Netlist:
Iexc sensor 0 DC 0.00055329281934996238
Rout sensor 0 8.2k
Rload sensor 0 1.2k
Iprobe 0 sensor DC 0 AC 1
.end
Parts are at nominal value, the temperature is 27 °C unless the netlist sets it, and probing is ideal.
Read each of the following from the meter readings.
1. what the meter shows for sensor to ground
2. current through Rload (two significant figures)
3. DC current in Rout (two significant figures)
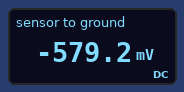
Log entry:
-579.2 mV
480 µA
71 µA
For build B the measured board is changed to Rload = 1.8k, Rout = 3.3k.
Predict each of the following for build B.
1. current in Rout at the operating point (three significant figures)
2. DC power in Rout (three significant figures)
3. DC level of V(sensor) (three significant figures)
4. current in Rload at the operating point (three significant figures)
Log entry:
195 µA
126 µW
-644 mV
358 µA
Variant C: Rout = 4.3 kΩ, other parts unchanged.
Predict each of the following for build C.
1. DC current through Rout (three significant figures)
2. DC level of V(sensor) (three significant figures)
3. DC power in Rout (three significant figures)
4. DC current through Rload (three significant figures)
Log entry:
121 µA
-519 mV
62.7 µW
433 µA
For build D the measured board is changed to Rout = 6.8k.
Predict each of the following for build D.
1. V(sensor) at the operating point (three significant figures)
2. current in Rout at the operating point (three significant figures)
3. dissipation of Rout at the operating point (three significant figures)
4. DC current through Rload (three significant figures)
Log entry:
-564 mV
83.0 µA
46.8 µW
470 µA
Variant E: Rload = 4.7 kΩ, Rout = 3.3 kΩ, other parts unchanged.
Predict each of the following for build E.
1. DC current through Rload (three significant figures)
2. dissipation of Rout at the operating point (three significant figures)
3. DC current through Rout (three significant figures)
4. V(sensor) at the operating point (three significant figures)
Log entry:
228 µA
349 µW
325 µA
-1.07 V
